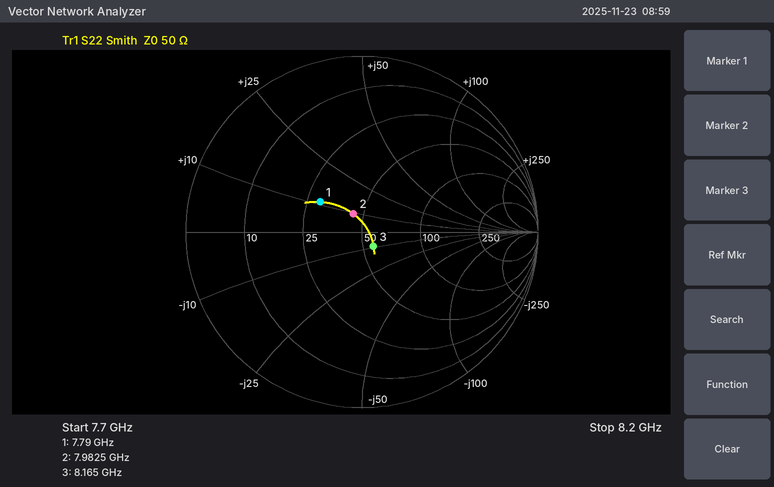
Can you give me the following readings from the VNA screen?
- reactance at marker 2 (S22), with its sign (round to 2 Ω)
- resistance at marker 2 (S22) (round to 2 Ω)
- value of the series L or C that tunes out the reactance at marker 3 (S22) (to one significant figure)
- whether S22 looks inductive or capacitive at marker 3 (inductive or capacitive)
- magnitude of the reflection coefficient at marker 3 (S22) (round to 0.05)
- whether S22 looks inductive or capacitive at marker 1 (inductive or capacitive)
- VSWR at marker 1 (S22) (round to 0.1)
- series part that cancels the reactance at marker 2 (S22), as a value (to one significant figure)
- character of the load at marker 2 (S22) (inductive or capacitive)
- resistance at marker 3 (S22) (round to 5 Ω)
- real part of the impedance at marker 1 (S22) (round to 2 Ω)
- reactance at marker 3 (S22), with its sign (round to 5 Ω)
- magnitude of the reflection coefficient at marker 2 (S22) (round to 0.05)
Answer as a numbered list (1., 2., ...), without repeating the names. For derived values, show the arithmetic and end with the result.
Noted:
1. +10 Ω
2. 44 Ω
3. L = 10 Ω/(2π × 8.165 GHz) ≈ 195 pH, so 200 pH to one significant figure
4. capacitive
5. 0.10
6. inductive
7. 1.8
8. C = 1/(2π × 7.9825 GHz × 10 Ω) ≈ 2 pF
9. inductive
10. 55 Ω
11. 30 Ω
12. -10 Ω
13. 0.10
